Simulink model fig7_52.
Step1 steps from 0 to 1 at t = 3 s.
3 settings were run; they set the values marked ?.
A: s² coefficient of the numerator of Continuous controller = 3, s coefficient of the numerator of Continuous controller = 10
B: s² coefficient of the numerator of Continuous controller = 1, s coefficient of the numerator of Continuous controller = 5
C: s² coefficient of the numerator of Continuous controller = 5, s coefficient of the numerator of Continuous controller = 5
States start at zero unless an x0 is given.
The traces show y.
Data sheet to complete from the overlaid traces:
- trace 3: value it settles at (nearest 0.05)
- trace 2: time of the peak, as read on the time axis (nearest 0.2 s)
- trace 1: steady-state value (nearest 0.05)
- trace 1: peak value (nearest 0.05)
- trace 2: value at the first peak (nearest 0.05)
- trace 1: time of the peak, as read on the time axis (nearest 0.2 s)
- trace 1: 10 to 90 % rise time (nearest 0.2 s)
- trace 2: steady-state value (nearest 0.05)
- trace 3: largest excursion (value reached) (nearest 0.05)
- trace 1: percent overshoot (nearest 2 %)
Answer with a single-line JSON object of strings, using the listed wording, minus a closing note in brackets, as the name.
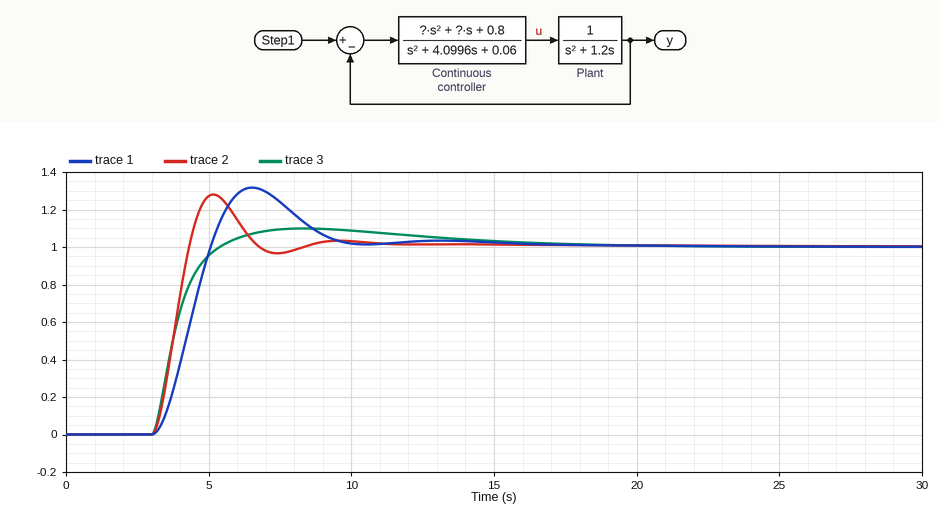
{"trace 3: value it settles at": "1.00", "trace 2: time of the peak, as read on the time axis": "5.2 s", "trace 1: steady-state value": "1.00", "trace 1: peak value": "1.30", "trace 2: value at the first peak": "1.30", "trace 1: time of the peak, as read on the time axis": "6.6 s", "trace 1: 10 to 90 % rise time": "1.4 s", "trace 2: steady-state value": "1.00", "trace 3: largest excursion (value reached)": "1.10", "trace 1: percent overshoot": "32 %"}
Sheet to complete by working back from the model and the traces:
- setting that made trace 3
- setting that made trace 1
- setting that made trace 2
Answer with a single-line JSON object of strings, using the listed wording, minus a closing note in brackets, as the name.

{"setting that made trace 3": "C", "setting that made trace 1": "B", "setting that made trace 2": "A"}
